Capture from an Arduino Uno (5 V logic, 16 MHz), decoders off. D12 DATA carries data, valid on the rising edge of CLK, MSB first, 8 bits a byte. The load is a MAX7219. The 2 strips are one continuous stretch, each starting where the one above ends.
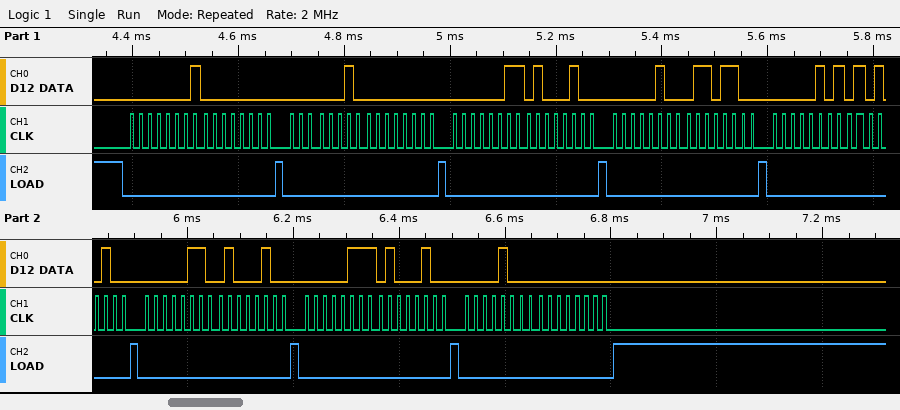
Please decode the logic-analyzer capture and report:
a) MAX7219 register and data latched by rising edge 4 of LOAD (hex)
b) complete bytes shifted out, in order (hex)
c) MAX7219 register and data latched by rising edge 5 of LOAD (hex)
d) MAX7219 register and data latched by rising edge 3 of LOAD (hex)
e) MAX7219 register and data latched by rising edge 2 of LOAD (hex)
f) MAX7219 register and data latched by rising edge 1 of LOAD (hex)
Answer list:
register 0x4, data 0x6C
01 00 02 00 03 44 04 6C 05 54 06 44 07 44 08 00
register 0x5, data 0x54
register 0x3, data 0x44
register 0x2, data 0x00
register 0x1, data 0x00
